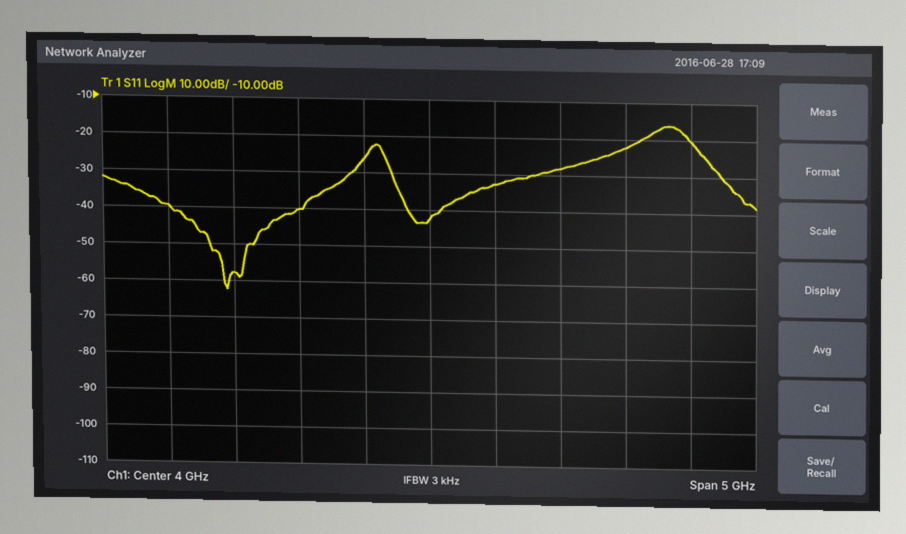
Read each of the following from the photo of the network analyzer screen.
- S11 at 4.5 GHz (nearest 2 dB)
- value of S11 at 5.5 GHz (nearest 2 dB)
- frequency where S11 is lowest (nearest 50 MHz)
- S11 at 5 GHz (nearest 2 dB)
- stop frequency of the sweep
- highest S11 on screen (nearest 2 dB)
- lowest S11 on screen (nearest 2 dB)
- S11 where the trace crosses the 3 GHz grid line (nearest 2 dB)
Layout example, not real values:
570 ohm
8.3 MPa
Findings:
-32 dB
-22 dB
2.45 GHz
-28 dB
6.5 GHz
-16 dB
-62 dB
-40 dB
